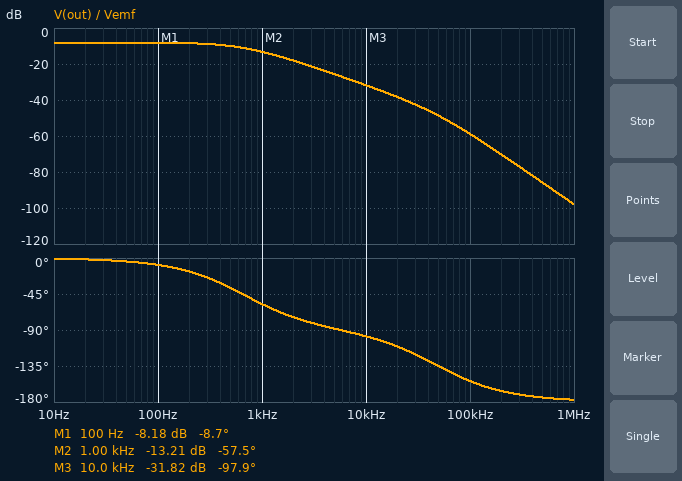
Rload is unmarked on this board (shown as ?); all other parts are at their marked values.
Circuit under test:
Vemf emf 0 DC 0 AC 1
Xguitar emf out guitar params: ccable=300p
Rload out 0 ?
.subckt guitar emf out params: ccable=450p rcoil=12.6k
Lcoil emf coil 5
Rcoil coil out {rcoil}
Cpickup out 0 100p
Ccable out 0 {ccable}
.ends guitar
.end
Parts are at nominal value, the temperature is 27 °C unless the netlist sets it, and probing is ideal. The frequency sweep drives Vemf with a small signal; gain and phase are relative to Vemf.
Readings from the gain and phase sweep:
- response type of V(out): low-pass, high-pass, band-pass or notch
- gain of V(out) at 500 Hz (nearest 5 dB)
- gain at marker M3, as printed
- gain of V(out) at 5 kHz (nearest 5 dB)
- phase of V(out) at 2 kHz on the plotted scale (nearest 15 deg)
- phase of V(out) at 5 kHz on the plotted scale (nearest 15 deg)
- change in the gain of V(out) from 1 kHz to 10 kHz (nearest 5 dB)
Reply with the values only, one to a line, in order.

low-pass
-10 dB
-31.82 dB
-25 dB
-75 deg
-90 deg
-20 dB
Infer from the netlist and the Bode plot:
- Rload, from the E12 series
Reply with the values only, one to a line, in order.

8.2 kΩ
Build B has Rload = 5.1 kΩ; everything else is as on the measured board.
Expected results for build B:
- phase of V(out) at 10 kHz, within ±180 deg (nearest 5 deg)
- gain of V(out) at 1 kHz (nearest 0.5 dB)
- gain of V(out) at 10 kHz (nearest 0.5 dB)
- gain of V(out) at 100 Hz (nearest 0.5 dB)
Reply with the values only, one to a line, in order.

-95 deg
-17.0 dB
-36.0 dB
-11.0 dB
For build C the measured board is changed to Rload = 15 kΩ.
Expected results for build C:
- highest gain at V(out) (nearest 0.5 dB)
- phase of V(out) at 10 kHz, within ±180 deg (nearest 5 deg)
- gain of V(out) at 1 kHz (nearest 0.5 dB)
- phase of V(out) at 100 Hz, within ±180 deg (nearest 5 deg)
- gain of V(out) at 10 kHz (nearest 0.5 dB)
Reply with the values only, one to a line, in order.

-5.5 dB
-105 deg
-9.0 dB
-5 deg
-27.0 dB
